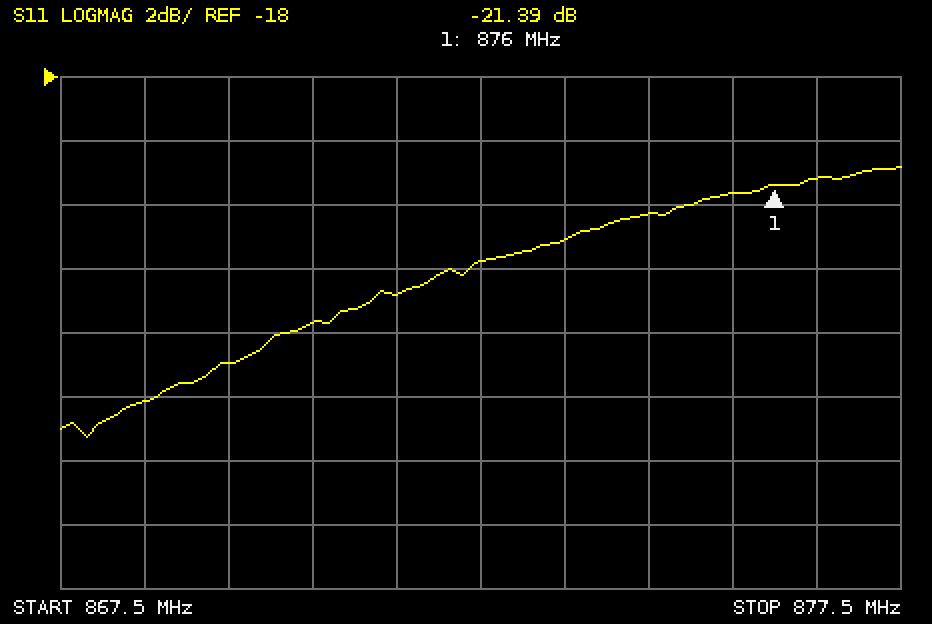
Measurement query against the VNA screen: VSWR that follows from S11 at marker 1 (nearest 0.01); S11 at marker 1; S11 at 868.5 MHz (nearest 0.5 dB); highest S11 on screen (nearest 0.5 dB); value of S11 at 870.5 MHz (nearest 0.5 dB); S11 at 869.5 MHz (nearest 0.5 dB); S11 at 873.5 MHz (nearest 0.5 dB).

1.19
-21.39 dB
-28.0 dB
-21.0 dB
-25.5 dB
-27.0 dB
-23.0 dB
